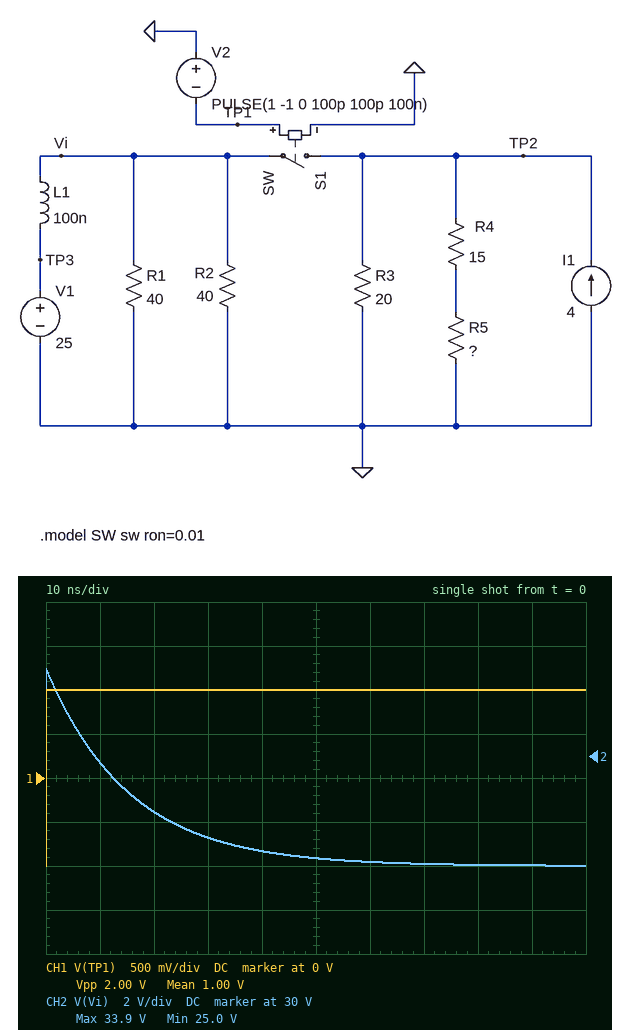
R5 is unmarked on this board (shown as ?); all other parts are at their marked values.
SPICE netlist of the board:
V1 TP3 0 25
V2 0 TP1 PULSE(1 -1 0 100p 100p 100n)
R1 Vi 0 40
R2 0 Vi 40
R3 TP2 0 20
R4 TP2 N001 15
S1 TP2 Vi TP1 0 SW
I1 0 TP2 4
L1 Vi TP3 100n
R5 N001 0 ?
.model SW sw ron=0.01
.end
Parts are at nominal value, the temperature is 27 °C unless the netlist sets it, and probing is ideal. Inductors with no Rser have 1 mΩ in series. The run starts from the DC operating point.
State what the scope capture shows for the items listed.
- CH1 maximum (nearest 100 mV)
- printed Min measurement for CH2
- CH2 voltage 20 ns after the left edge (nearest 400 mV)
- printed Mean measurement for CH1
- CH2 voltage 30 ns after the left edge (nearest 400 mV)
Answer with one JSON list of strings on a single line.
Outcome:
["1.0 V", "25.0 V", "27.6 V", "1.00 V", "26.4 V"]
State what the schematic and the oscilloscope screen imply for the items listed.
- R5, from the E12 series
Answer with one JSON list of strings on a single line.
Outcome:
["3.3 Ω"]
